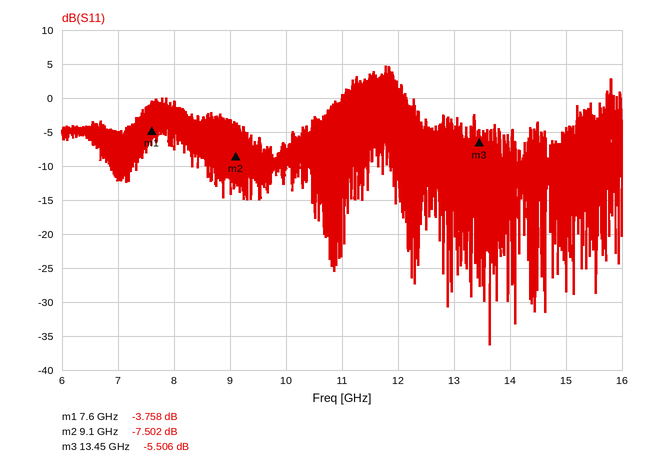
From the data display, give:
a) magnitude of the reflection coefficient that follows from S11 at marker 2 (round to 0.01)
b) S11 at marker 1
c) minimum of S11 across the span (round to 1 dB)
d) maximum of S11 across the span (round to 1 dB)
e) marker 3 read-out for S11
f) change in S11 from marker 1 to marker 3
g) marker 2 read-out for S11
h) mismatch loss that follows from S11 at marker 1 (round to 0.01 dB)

0.42
-3.758 dB
-36 dB
5 dB
-5.506 dB
-1.748 dB
-7.502 dB
2.37 dB
